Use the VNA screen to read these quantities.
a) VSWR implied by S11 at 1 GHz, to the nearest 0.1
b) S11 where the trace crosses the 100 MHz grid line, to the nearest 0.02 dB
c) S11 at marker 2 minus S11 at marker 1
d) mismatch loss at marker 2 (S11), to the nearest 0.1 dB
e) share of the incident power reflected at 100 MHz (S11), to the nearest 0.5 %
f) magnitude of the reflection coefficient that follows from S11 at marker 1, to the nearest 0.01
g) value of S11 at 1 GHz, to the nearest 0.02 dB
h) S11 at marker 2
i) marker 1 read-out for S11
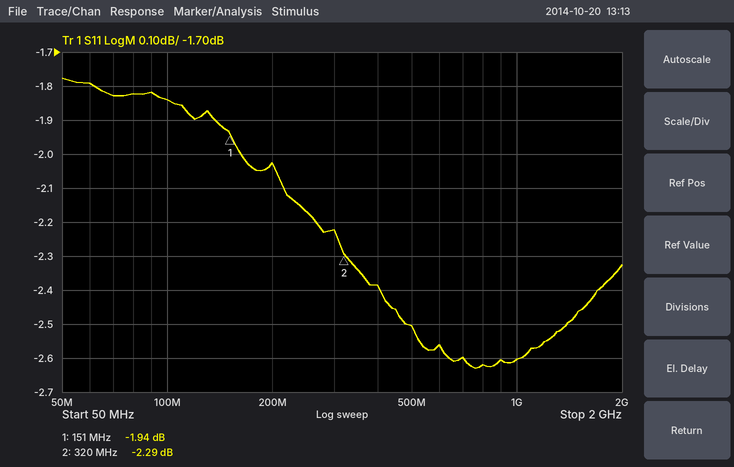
6.7
-1.84 dB
-0.35 dB
3.9 dB
65.5 %
0.80
-2.60 dB
-2.29 dB
-1.94 dB
